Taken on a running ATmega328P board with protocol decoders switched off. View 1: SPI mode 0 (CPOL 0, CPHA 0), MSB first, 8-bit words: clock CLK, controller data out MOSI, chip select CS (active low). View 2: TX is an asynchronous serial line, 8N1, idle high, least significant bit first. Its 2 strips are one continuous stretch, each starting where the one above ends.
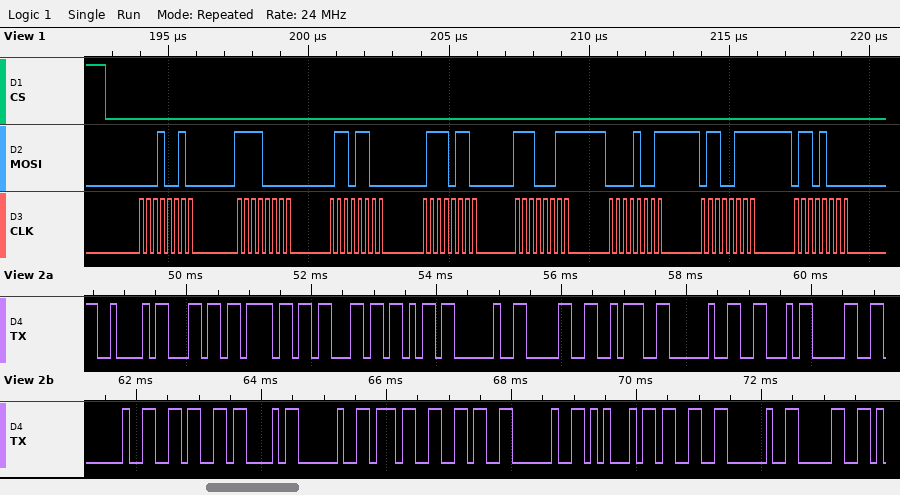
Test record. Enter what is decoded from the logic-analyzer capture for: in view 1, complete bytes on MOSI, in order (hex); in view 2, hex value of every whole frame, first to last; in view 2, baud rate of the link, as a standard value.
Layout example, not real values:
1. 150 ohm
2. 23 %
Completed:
1. 12 F0 6C 76 E3 09 67 68
2. 42 6C 6F 63 6B 20 30 3A 20 46 30 20 36 43 20 37 36 20 45 33 20 30
3. 9600 baud
